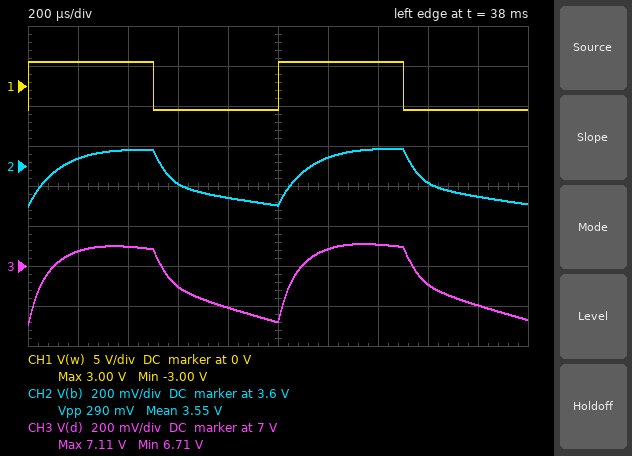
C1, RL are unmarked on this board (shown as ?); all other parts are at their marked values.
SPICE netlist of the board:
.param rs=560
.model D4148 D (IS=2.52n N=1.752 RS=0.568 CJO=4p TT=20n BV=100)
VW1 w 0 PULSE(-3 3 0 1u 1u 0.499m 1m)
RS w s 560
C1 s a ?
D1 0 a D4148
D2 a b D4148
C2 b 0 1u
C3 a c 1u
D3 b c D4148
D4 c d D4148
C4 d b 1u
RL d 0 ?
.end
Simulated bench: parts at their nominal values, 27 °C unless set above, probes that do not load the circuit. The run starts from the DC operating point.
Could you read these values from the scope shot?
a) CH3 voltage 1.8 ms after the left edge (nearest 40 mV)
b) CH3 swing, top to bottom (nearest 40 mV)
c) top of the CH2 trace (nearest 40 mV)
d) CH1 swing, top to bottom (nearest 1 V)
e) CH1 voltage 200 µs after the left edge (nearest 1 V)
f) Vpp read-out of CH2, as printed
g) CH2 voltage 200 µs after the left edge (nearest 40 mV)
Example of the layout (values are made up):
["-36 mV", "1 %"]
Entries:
["6.80 V", "400 mV", "3.68 V", "6 V", "3 V", "290 mV", "3.64 V"]
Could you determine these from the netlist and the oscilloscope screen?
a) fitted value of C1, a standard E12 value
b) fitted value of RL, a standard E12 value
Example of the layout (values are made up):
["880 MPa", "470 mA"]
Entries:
["330 nF", "39 kΩ"]
